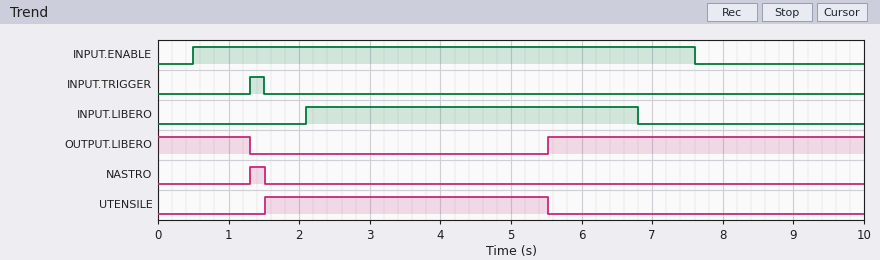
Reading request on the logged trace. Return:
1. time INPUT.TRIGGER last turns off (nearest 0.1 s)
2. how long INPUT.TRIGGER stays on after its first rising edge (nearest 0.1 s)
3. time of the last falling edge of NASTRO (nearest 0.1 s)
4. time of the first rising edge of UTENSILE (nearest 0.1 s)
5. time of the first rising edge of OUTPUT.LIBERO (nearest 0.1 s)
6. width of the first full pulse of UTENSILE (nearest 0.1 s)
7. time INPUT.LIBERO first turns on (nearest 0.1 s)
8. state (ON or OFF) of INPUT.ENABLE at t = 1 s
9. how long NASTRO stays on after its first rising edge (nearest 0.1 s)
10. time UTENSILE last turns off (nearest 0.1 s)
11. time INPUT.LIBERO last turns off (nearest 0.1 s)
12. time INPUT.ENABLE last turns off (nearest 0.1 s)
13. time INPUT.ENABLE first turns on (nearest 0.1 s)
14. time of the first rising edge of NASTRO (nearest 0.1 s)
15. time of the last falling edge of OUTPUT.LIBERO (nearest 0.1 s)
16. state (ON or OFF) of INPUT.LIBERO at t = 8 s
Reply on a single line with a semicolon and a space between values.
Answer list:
1.5 s; 0.2 s; 1.5 s; 1.5 s; 5.5 s; 4.0 s; 2.1 s; ON; 0.2 s; 5.5 s; 6.8 s; 7.6 s; 0.5 s; 1.3 s; 1.3 s; OFF
